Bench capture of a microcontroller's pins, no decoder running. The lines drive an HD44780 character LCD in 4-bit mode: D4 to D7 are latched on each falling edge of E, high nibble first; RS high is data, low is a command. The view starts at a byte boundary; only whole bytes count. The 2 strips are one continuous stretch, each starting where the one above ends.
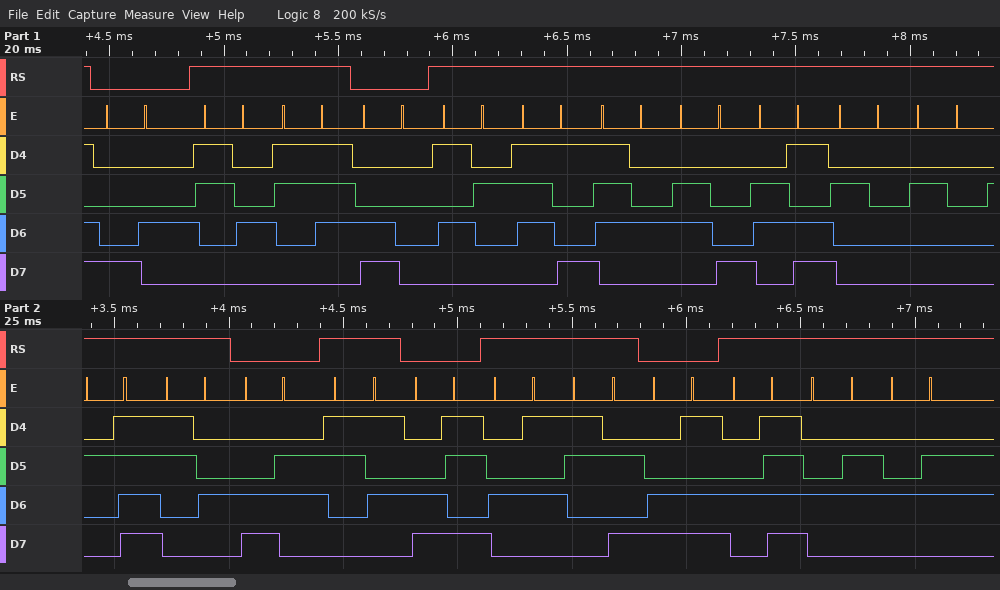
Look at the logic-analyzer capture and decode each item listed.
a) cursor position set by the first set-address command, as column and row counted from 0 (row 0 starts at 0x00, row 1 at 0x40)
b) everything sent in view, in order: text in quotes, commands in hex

column 4, row 0
0x84 "47" 0xC0 "Rythm  /4" 0xC6 "5" 0xCB "E:" 0xCD "OFF"
